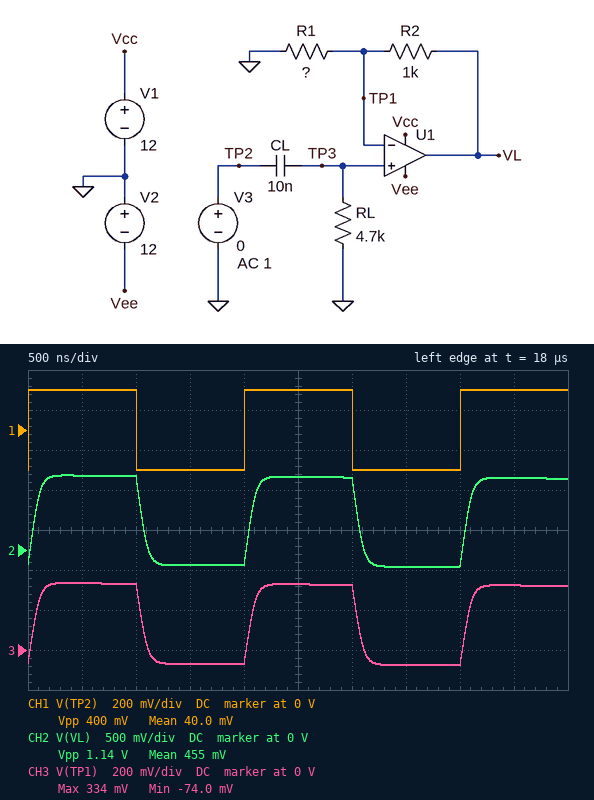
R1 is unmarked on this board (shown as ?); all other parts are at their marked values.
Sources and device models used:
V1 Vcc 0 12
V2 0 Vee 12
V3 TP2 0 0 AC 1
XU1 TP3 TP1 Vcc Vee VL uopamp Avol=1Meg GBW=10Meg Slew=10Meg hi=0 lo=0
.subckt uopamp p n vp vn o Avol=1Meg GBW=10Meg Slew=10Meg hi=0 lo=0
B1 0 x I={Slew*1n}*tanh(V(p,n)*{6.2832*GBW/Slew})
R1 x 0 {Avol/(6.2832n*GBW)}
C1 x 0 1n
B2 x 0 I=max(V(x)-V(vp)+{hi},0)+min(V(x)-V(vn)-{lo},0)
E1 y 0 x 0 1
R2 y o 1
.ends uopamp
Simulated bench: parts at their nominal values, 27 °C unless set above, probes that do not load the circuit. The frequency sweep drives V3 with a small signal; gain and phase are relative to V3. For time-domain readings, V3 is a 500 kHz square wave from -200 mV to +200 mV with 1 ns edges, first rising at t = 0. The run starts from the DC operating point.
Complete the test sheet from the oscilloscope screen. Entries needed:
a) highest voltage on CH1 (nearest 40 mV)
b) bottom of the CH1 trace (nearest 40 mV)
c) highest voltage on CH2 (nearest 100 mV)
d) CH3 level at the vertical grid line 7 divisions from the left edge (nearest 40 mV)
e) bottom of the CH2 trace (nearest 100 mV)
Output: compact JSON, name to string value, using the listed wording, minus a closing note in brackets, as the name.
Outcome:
{"highest voltage on CH1": "200 mV", "bottom of the CH1 trace": "-200 mV", "highest voltage on CH2": "900 mV", "CH3 level at the vertical grid line 7 divisions from the left edge": "-80 mV", "bottom of the CH2 trace": "-200 mV"}
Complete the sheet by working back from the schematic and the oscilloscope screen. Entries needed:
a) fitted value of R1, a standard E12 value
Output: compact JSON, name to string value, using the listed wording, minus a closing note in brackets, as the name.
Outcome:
{"fitted value of R1, a standard E12 value": "560 Ω"}
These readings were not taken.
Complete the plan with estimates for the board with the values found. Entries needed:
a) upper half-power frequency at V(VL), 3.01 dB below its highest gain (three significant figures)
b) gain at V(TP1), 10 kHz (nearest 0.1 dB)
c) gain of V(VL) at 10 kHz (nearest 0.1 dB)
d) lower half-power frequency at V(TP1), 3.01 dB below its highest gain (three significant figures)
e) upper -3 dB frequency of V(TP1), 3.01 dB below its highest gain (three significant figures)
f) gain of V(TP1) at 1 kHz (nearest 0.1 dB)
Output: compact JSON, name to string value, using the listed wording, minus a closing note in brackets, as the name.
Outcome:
{"upper half-power frequency at V(VL), 3.01 dB below its highest gain": "3.59 MHz", "gain at V(TP1), 10 kHz": "-0.5 dB", "gain of V(VL) at 10 kHz": "8.4 dB", "lower half-power frequency at V(TP1), 3.01 dB below its highest gain": "3.38 kHz", "upper -3 dB frequency of V(TP1), 3.01 dB below its highest gain": "3.59 MHz", "gain of V(TP1) at 1 kHz": "-11.0 dB"}
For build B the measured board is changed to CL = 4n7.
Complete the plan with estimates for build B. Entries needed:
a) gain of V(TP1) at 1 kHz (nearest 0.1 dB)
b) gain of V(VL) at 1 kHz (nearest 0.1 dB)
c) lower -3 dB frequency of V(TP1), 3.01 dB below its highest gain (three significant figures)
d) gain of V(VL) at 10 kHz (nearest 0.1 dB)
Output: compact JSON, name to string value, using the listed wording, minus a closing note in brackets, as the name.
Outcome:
{"gain of V(TP1) at 1 kHz": "-17.2 dB", "gain of V(VL) at 1 kHz": "-8.3 dB", "lower -3 dB frequency of V(TP1), 3.01 dB below its highest gain": "7.18 kHz", "gain of V(VL) at 10 kHz": "7.1 dB"}
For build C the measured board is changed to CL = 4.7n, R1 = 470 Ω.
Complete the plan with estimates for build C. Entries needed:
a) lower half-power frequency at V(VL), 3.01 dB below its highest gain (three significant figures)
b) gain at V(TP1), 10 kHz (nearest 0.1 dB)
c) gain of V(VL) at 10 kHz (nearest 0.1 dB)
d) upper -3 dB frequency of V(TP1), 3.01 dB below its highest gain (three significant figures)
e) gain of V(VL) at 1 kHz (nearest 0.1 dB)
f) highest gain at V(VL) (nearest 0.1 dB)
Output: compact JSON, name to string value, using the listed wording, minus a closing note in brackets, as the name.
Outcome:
{"lower half-power frequency at V(VL), 3.01 dB below its highest gain": "7.17 kHz", "gain at V(TP1), 10 kHz": "-1.8 dB", "gain of V(VL) at 10 kHz": "8.1 dB", "upper -3 dB frequency of V(TP1), 3.01 dB below its highest gain": "3.21 MHz", "gain of V(VL) at 1 kHz": "-7.3 dB", "highest gain at V(VL)": "9.9 dB"}
